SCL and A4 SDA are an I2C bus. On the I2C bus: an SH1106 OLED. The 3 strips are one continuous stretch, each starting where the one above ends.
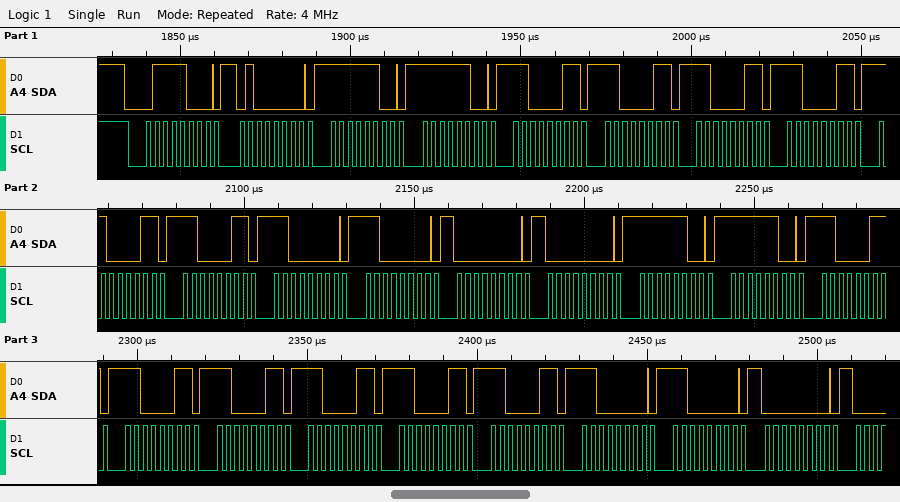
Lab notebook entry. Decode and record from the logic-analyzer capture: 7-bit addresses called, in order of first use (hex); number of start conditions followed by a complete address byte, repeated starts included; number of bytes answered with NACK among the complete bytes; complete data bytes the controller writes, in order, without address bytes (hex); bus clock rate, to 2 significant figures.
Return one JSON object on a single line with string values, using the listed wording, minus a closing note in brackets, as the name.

{"7-bit addresses called, in order of first use": "0x3C", "number of start conditions followed by a complete address byte, repeated starts included": "1", "number of bytes answered with NACK among the complete bytes": "0", "complete data bytes the controller writes, in order, without address bytes": "40 FC FC C3 C3 C3 C3 C3 C3 C0 C0 00 00 FC FC C3 C3 C3 C3 C3 C3 C0 C0 00", "bus clock rate, to 2 significant figures": "400 kHz"}
